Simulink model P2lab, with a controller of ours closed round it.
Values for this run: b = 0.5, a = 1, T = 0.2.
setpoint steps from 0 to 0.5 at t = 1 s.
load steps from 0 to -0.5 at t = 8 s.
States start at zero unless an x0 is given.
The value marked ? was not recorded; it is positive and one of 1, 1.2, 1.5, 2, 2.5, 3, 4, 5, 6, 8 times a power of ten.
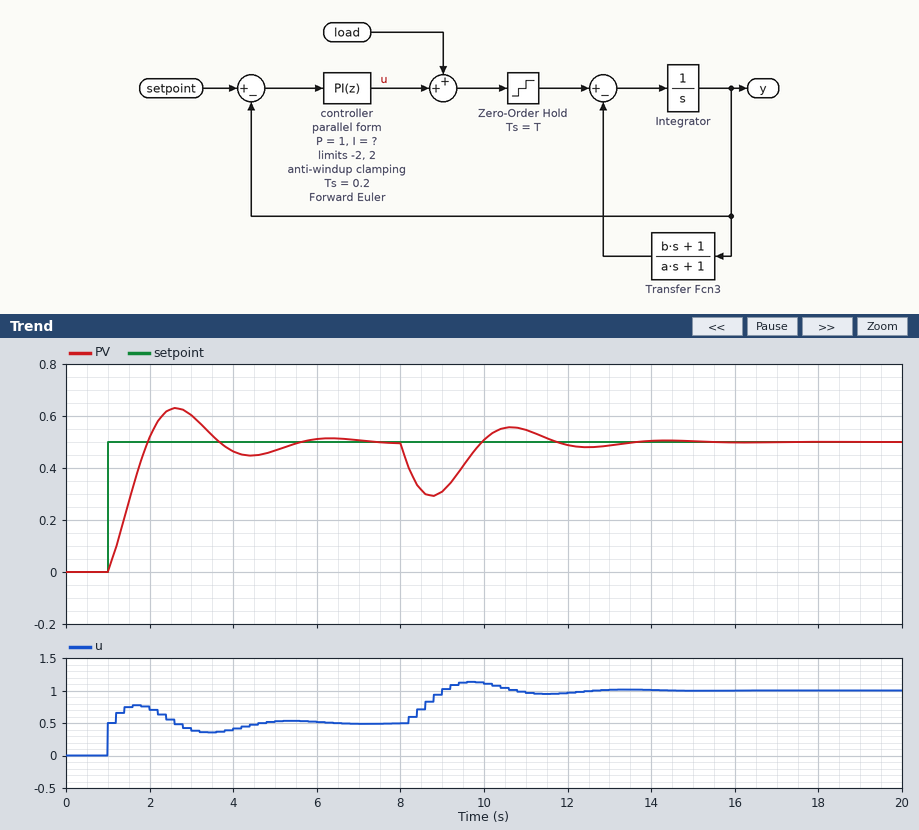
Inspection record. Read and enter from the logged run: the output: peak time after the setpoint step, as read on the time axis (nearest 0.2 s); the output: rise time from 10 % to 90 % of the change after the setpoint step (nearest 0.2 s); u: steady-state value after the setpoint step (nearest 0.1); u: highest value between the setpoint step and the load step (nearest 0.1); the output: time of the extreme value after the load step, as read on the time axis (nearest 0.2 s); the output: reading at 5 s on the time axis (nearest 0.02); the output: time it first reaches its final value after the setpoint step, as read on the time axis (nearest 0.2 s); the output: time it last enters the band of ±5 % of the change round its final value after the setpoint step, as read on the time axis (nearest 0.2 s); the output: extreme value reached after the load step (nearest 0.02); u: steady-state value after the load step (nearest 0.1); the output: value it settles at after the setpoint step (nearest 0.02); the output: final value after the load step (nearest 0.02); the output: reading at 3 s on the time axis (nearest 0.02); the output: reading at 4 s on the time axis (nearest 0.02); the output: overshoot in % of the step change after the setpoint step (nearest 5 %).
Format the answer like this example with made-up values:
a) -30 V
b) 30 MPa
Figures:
a) 2.6 s
b) 0.8 s
c) 0.5
d) 0.8
e) 8.8 s
f) 0.46
g) 2.0 s
h) 5.2 s
i) 0.30
j) 1.0
k) 0.50
l) 0.50
m) 0.60
n) 0.46
o) 25 %
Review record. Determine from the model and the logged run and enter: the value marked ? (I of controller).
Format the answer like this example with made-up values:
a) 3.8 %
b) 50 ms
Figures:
a) 2.5
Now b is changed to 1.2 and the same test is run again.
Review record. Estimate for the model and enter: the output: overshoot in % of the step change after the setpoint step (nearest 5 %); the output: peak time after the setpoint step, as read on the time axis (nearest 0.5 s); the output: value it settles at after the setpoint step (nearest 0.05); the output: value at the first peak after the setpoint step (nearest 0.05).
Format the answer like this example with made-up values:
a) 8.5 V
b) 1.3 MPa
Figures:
a) 20 %
b) 3.0 s
c) 0.50
d) 0.60
